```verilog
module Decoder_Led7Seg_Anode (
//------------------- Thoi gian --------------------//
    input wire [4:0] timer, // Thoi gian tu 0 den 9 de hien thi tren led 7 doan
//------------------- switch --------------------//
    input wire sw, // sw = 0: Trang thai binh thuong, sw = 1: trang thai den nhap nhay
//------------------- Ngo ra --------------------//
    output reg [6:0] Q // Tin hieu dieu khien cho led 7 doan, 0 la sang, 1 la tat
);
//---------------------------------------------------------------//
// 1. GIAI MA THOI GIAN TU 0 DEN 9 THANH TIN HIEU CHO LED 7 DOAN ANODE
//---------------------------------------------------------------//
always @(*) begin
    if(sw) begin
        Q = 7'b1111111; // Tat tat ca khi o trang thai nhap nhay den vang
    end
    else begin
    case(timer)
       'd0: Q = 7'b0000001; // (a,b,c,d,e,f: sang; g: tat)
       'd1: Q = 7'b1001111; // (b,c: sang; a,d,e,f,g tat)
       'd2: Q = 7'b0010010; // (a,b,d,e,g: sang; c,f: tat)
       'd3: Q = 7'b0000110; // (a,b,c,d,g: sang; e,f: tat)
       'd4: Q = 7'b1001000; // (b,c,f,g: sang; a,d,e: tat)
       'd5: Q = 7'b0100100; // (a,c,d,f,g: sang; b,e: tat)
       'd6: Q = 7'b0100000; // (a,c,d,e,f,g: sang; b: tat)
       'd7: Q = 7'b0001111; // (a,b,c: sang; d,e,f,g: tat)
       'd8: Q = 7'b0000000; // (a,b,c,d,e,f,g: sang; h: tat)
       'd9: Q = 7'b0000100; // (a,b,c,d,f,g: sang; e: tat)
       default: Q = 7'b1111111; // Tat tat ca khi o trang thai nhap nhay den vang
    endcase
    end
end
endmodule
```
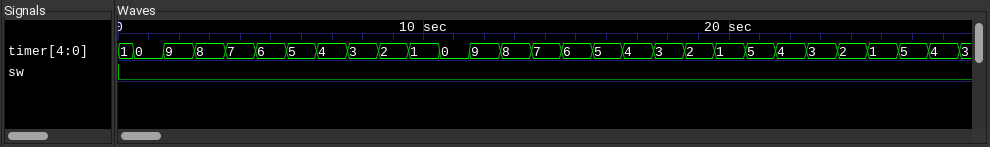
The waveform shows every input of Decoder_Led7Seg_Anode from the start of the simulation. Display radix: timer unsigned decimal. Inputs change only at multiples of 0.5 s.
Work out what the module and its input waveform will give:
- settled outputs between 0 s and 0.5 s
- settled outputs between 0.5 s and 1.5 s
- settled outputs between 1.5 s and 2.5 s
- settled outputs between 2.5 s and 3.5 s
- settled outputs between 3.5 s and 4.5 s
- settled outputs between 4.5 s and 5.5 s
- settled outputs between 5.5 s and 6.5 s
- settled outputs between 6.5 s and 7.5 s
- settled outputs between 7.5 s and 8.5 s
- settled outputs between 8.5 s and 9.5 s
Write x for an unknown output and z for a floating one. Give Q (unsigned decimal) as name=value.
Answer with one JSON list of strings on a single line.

["Q=79", "Q=1", "Q=4", "Q=0", "Q=15", "Q=32", "Q=36", "Q=72", "Q=6", "Q=18"]
